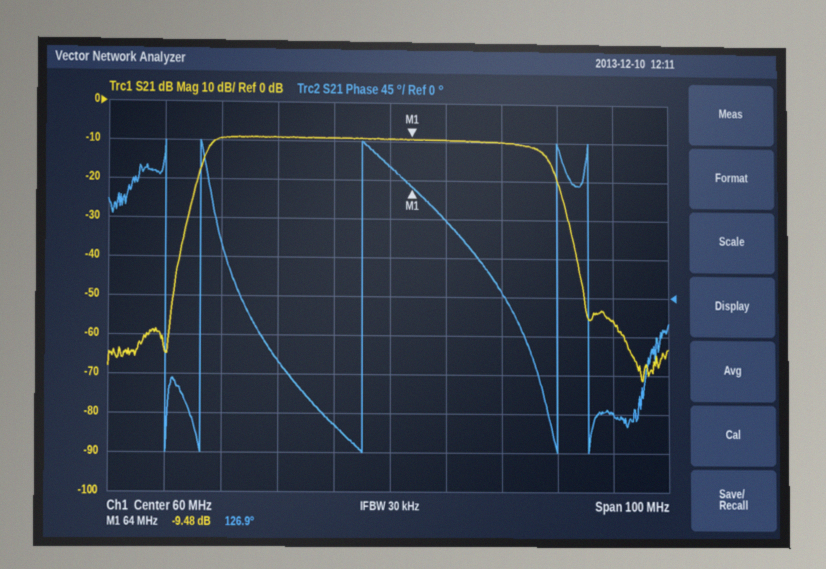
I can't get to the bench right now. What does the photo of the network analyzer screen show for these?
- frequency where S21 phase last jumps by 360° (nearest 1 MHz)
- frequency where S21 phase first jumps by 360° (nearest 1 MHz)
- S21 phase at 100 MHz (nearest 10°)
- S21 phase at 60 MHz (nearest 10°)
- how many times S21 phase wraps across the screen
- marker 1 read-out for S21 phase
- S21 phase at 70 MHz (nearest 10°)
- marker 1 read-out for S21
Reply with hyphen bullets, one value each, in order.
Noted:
- 96 MHz
- 20 MHz
- -130°
- 150°
- 5
- 126.9°
- 90°
- -9.48 dB
